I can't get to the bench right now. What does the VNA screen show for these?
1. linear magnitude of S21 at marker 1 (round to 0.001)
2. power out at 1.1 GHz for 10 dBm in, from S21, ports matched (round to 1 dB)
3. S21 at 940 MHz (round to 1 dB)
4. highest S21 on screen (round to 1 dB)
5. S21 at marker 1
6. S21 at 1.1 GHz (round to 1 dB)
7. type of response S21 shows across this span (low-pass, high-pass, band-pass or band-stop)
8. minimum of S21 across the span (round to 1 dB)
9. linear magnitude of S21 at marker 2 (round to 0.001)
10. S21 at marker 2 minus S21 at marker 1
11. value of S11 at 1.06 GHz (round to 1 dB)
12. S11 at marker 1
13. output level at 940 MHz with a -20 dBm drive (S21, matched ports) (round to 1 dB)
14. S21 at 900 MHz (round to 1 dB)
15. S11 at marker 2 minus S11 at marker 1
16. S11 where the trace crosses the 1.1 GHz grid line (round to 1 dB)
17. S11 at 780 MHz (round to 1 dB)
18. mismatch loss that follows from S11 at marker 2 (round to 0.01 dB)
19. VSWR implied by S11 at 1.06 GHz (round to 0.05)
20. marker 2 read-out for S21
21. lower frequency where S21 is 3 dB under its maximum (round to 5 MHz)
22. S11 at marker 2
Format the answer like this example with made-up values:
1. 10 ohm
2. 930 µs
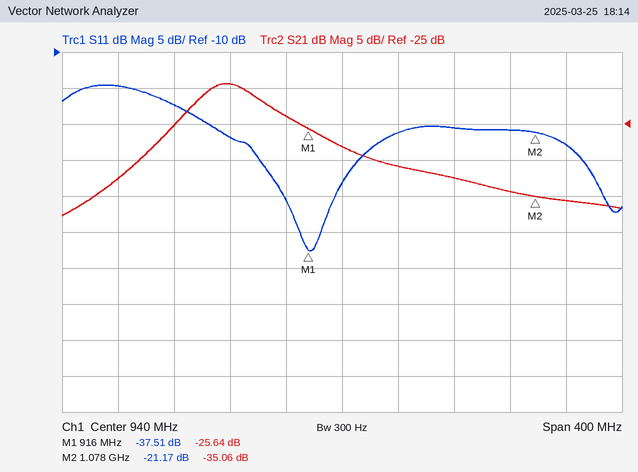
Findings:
1. 0.052
2. -26 dBm
3. -28 dB
4. -19 dB
5. -25.64 dB
6. -36 dB
7. band-pass
8. -38 dB
9. 0.018
10. -9.42 dB
11. -21 dB
12. -37.51 dB
13. -48 dBm
14. -24 dB
15. 16.34 dB
16. -23 dB
17. -15 dB
18. 0.03 dB
19. 1.20
20. -35.06 dB
21. 835 MHz
22. -21.17 dB
